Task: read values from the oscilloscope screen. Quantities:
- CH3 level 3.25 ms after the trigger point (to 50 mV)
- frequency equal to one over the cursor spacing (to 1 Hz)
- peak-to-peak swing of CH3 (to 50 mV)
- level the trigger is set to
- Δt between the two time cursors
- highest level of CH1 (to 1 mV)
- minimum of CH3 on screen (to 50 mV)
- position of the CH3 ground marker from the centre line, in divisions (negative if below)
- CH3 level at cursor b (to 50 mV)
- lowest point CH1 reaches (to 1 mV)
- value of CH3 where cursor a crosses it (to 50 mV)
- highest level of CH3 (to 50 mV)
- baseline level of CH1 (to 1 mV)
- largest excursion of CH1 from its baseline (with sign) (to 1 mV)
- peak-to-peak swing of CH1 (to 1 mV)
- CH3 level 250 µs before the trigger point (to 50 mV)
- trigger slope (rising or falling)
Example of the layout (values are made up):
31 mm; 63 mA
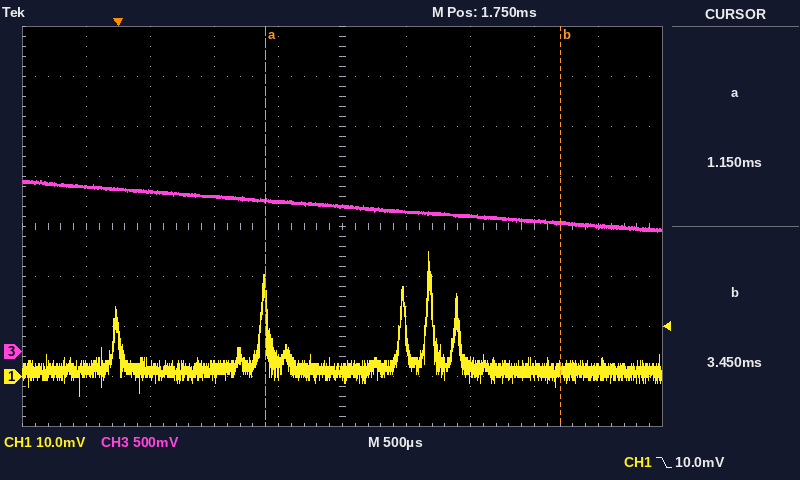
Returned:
1.30 V; 435 Hz; 500 mV; 10.0 mV; 2.30 ms; 25 mV; 1.20 V; -2.5 div; 1.30 V; -4 mV; 1.50 V; 1.70 V; 1 mV; +24 mV; 29 mV; 1.65 V; falling
